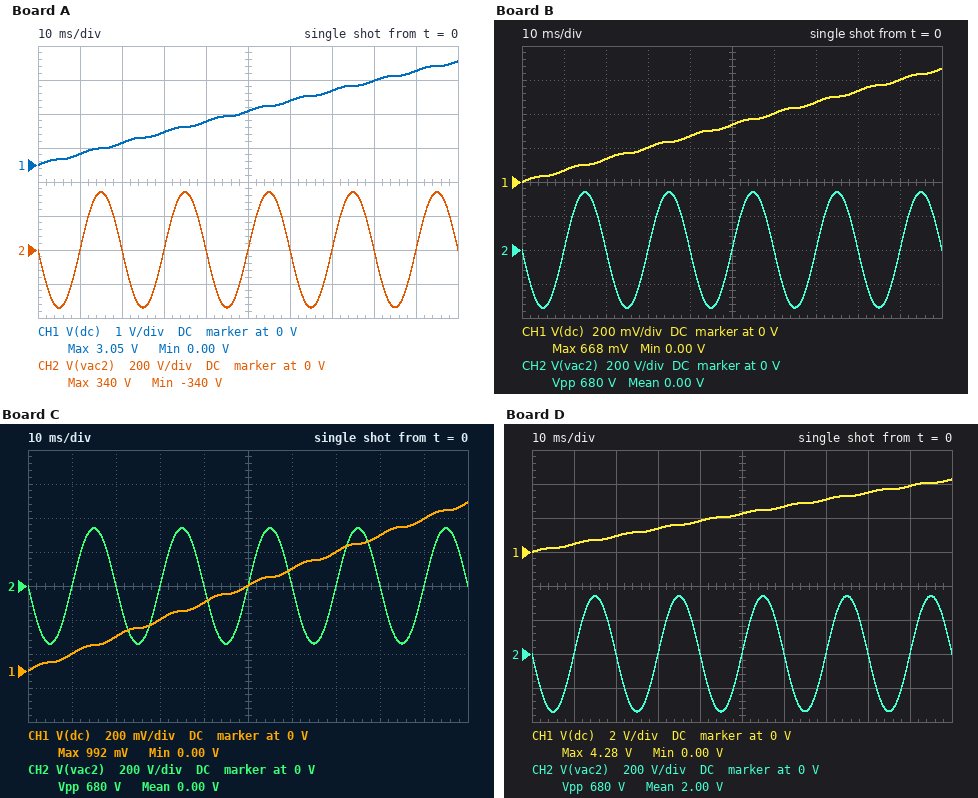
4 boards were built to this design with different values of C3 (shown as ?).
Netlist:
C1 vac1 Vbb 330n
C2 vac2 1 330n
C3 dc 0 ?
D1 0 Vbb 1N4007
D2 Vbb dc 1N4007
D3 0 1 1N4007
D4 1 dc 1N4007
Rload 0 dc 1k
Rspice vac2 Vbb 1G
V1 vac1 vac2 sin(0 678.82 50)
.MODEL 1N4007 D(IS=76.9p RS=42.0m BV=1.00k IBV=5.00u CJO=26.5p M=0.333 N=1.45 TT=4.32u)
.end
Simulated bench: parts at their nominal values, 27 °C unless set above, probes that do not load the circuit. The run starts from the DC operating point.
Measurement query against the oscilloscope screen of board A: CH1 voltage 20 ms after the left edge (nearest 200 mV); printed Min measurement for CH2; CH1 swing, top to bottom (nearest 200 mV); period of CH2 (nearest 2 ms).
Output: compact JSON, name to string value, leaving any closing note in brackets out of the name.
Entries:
{"CH1 voltage 20 ms after the left edge": "600 mV", "printed Min measurement for CH2": "-340 V", "CH1 swing, top to bottom": "3.0 V", "period of CH2": "20 ms"}
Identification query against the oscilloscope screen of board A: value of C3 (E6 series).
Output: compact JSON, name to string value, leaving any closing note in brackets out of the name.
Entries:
{"value of C3": "680 µF"}
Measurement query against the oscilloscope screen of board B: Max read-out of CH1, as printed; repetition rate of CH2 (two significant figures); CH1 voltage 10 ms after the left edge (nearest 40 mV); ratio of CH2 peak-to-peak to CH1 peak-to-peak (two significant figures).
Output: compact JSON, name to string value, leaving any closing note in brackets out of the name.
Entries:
{"Max read-out of CH1, as printed": "668 mV", "repetition rate of CH2": "50 Hz", "CH1 voltage 10 ms after the left edge": "80 mV", "ratio of CH2 peak-to-peak to CH1 peak-to-peak": "1000"}
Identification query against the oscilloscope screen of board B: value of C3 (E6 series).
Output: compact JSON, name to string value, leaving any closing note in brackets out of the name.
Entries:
{"value of C3": "3.3 mF"}
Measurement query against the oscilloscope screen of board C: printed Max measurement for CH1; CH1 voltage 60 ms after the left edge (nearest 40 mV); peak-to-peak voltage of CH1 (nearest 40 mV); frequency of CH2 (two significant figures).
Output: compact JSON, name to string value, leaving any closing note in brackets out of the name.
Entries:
{"printed Max measurement for CH1": "992 mV", "CH1 voltage 60 ms after the left edge": "600 mV", "peak-to-peak voltage of CH1": "1.00 V", "frequency of CH2": "50 Hz"}
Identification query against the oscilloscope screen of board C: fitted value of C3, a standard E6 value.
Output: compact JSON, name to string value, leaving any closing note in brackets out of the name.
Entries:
{"fitted value of C3, a standard E6 value": "2.2 mF"}
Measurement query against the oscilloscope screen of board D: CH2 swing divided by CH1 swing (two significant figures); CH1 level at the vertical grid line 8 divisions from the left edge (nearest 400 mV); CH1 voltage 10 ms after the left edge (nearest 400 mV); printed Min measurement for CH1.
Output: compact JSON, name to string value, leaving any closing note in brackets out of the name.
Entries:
{"CH2 swing divided by CH1 swing": "160", "CH1 level at the vertical grid line 8 divisions from the left edge": "3.6 V", "CH1 voltage 10 ms after the left edge": "400 mV", "printed Min measurement for CH1": "0.00 V"}
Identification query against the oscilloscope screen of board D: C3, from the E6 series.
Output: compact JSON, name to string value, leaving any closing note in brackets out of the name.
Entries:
{"C3, from the E6 series": "470 µF"}
